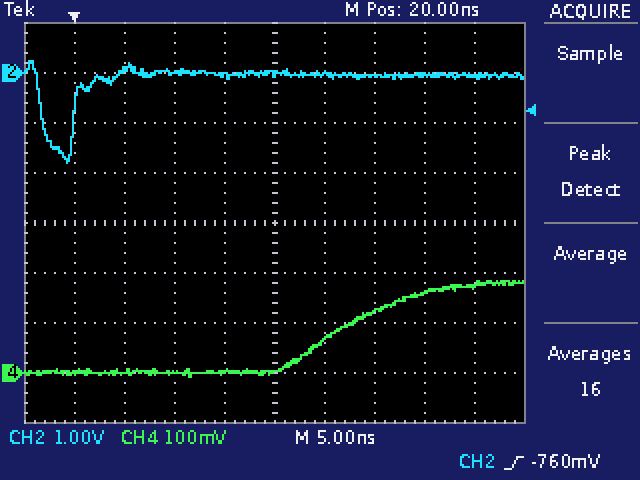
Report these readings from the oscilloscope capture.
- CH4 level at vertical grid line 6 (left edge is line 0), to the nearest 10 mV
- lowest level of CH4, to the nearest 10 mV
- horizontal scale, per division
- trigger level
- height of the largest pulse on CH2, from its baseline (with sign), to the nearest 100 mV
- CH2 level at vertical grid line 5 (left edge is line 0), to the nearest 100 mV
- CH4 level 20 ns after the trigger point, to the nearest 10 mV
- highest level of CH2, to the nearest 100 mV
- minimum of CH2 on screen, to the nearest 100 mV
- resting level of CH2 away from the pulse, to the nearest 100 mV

70 mV
-10 mV
5 ns
-760 mV
-1.8 V
0.0 V
0 mV
200 mV
-1.8 V
0.0 V
